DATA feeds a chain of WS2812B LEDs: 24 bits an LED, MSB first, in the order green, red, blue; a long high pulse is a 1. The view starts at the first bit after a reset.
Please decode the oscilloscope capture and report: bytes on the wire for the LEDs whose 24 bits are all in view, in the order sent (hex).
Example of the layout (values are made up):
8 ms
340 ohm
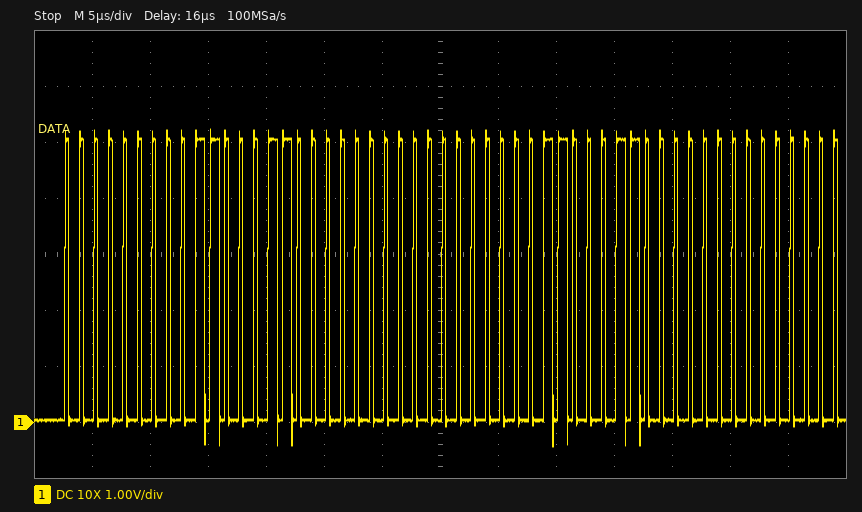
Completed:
00 63 00 00 63 00
